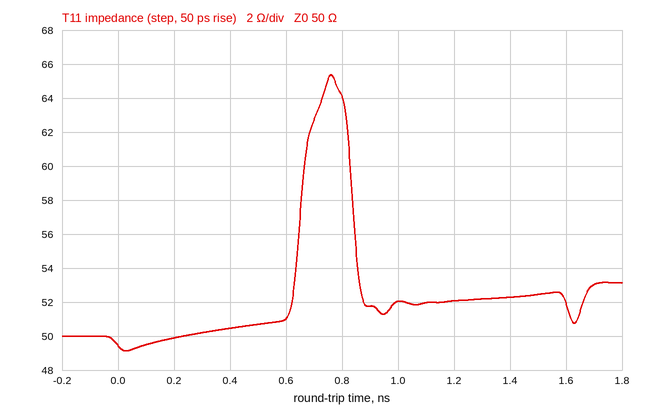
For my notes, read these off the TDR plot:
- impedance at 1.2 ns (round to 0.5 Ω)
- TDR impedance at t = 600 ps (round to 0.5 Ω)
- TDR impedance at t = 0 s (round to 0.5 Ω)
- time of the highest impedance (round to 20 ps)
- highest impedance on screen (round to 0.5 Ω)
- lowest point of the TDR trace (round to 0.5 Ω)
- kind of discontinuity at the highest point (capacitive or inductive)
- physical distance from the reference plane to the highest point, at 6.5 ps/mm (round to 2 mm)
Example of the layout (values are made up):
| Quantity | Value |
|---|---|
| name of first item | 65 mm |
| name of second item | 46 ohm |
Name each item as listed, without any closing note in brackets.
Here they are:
| Quantity | Value |
|---|---|
| impedance at 1.2 ns | 52.0 Ω |
| TDR impedance at t = 600 ps | 51.0 Ω |
| TDR impedance at t = 0 s | 49.5 Ω |
| time of the highest impedance | 760 ps |
| highest impedance on screen | 65.5 Ω |
| lowest point of the TDR trace | 49.0 Ω |
| kind of discontinuity at the highest point | inductive |
| physical distance from the reference plane to the highest point, at 6.5 ps/mm | 58 mm |
